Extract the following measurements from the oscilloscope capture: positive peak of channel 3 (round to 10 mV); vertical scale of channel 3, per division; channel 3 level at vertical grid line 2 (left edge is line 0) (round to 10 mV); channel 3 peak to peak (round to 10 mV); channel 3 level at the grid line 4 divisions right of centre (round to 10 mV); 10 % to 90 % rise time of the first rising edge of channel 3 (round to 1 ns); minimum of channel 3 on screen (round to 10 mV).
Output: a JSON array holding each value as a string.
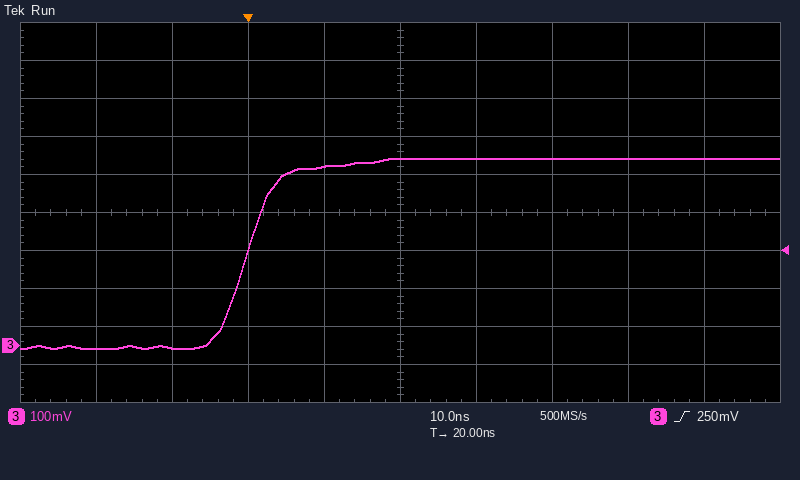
["490 mV", "100 mV", "-10 mV", "500 mV", "490 mV", "8 ns", "-10 mV"]
